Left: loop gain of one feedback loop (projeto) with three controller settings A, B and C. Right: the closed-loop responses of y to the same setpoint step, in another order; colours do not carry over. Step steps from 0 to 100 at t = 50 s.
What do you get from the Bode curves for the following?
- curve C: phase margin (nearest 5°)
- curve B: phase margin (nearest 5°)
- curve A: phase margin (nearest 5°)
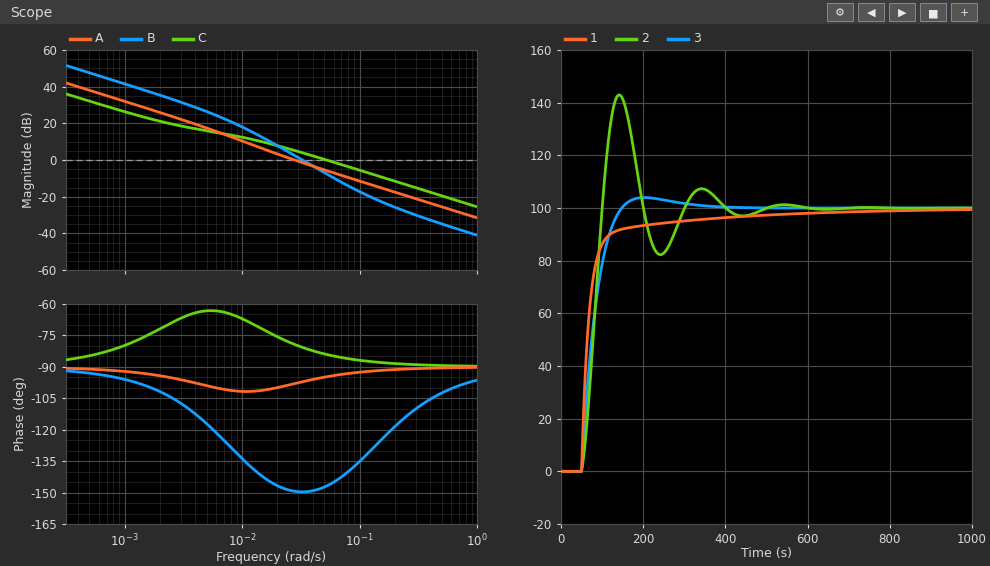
95°
30°
80°
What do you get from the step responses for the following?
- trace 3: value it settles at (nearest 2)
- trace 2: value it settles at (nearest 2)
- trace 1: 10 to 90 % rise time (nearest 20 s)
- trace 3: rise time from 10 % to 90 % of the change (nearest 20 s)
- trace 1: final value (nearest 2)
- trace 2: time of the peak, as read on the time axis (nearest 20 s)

100
100
60 s
60 s
100
140 s
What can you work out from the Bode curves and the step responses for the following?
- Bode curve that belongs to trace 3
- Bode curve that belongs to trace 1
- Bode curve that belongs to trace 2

A
C
B
